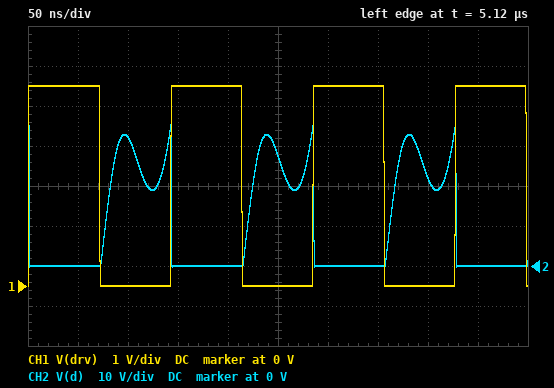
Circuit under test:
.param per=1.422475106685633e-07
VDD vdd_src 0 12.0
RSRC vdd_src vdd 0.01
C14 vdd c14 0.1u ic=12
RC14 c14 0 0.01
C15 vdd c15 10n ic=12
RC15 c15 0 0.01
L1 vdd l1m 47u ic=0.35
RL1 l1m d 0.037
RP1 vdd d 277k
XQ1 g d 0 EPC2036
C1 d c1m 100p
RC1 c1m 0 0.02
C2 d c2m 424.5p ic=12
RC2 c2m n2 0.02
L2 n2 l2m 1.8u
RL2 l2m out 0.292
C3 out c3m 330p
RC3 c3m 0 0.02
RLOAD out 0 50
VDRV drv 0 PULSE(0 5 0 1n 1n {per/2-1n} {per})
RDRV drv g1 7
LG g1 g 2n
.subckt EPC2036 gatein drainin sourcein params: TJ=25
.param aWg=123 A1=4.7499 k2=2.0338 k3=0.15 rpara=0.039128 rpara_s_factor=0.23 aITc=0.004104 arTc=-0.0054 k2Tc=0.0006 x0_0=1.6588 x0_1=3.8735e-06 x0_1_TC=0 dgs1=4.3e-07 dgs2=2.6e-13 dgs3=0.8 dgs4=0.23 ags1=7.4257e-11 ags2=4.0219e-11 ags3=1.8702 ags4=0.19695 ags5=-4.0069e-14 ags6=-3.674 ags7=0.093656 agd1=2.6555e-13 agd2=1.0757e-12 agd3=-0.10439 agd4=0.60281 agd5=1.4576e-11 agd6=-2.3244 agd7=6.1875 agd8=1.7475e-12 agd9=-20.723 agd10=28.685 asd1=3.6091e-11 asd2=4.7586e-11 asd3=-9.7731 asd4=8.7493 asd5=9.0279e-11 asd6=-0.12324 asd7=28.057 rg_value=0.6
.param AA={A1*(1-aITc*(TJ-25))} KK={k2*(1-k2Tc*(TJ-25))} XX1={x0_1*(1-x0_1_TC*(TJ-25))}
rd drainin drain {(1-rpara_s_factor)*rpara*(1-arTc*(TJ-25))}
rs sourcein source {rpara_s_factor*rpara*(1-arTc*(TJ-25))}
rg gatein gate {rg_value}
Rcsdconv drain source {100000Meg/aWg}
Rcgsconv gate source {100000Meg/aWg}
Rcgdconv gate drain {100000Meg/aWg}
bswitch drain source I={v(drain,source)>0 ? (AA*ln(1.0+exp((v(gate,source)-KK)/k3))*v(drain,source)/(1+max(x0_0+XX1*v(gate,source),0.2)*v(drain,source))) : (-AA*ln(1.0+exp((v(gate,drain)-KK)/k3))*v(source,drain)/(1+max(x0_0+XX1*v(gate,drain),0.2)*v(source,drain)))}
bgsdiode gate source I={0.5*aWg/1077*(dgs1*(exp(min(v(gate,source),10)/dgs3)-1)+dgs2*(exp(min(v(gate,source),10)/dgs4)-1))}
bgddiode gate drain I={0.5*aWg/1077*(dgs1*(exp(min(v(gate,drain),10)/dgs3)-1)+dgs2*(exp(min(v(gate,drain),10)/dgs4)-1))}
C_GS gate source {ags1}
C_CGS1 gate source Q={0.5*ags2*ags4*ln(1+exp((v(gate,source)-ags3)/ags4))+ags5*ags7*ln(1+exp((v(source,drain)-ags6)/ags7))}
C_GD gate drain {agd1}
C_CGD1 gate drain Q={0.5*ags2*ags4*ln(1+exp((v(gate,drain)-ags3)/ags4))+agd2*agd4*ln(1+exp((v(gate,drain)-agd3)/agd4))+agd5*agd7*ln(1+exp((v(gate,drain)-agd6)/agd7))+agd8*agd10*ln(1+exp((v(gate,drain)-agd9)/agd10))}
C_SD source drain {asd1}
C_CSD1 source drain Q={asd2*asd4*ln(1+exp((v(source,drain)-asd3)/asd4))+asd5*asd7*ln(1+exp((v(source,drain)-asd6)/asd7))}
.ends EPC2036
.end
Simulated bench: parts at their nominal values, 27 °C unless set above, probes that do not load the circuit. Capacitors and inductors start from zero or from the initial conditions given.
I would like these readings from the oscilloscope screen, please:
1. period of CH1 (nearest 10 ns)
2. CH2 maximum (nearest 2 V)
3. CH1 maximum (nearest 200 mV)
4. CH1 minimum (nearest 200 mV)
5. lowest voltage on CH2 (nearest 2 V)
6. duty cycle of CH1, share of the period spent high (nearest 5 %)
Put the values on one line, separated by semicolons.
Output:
140 ns; 36 V; 5.0 V; 0 V; 0 V; 50 %
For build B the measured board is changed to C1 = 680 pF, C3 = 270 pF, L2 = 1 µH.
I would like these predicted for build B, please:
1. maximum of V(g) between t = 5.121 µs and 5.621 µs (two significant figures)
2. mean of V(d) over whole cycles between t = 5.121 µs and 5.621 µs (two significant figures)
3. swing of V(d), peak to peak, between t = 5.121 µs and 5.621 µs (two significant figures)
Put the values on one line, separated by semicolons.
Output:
5.0 V; 11 V; 43 V
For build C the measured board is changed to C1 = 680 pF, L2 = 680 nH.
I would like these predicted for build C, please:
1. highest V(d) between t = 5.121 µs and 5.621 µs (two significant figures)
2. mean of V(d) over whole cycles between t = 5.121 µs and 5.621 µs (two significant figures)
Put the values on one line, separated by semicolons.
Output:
40 V; 11 V
